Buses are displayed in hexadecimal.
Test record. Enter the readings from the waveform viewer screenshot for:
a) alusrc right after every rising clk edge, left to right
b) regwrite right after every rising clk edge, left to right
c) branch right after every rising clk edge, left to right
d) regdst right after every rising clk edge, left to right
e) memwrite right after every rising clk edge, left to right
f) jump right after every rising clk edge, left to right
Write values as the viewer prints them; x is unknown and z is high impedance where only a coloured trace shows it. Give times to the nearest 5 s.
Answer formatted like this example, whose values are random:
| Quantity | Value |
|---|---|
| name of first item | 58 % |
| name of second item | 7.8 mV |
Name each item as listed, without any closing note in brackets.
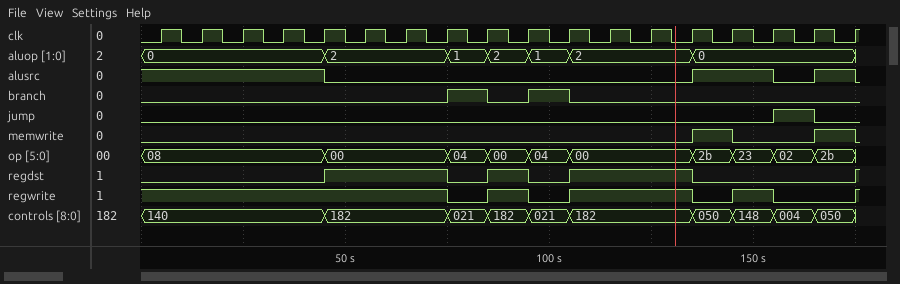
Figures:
| Quantity | Value |
|---|---|
| alusrc right after every rising clk edge, left to right | 1 1 1 1 0 0 0 0 0 0 0 0 0 1 1 0 1 0 |
| regwrite right after every rising clk edge, left to right | 1 1 1 1 1 1 1 0 1 0 1 1 1 0 1 0 0 1 |
| branch right after every rising clk edge, left to right | 0 0 0 0 0 0 0 1 0 1 0 0 0 0 0 0 0 0 |
| regdst right after every rising clk edge, left to right | 0 0 0 0 1 1 1 0 1 0 1 1 1 0 0 0 0 1 |
| memwrite right after every rising clk edge, left to right | 0 0 0 0 0 0 0 0 0 0 0 0 0 1 0 0 1 0 |
| jump right after every rising clk edge, left to right | 0 0 0 0 0 0 0 0 0 0 0 0 0 0 0 1 0 0 |
